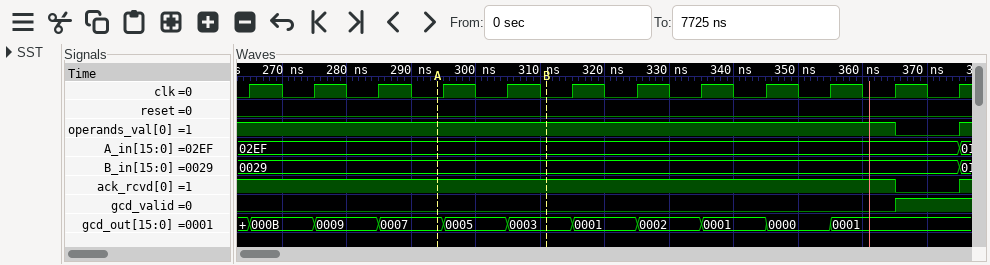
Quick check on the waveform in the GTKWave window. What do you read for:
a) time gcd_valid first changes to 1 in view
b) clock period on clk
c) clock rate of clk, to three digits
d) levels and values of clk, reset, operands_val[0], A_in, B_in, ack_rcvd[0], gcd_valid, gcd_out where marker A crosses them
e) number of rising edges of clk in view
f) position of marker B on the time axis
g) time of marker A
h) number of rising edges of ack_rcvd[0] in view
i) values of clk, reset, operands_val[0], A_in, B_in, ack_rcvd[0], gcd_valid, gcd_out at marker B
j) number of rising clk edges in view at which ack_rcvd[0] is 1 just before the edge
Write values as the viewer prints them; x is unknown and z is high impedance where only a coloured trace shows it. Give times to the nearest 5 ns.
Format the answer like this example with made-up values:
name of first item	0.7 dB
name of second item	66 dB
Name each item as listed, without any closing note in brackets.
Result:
time gcd_valid first changes to 1 in view	365 ns
clock period on clk	10 ns
clock rate of clk, to three digits	100 MHz
levels and values of clk, reset, operands_val[0], A_in, B_in, ack_rcvd[0], gcd_valid, gcd_out where marker A crosses them	clk=0, reset=0, operands_val[0]=1, A_in=02EF, B_in=0029, ack_rcvd[0]=1, gcd_valid=0, gcd_out=0007
number of rising edges of clk in view	12
position of marker B on the time axis	310 ns
time of marker A	295 ns
number of rising edges of ack_rcvd[0] in view	1
values of clk, reset, operands_val[0], A_in, B_in, ack_rcvd[0], gcd_valid, gcd_out at marker B	clk=0, reset=0, operands_val[0]=1, A_in=02EF, B_in=0029, ack_rcvd[0]=1, gcd_valid=0, gcd_out=0003
number of rising clk edges in view at which ack_rcvd[0] is 1 just before the edge	11
